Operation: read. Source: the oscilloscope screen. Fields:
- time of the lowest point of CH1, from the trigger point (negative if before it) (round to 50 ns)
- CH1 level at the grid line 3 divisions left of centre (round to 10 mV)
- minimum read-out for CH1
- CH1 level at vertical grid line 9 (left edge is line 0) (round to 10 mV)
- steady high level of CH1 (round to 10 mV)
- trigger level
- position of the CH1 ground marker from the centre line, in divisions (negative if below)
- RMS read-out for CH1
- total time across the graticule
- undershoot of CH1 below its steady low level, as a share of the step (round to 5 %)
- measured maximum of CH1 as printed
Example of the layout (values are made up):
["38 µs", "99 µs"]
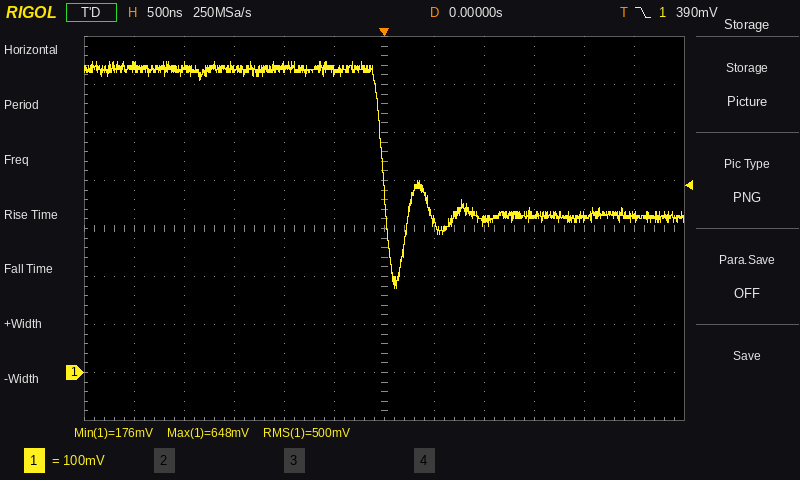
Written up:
["+100 ns", "630 mV", "176 mV", "330 mV", "630 mV", "390 mV", "-3.0 div", "500 mV", "6 µs", "50 %", "648 mV"]
